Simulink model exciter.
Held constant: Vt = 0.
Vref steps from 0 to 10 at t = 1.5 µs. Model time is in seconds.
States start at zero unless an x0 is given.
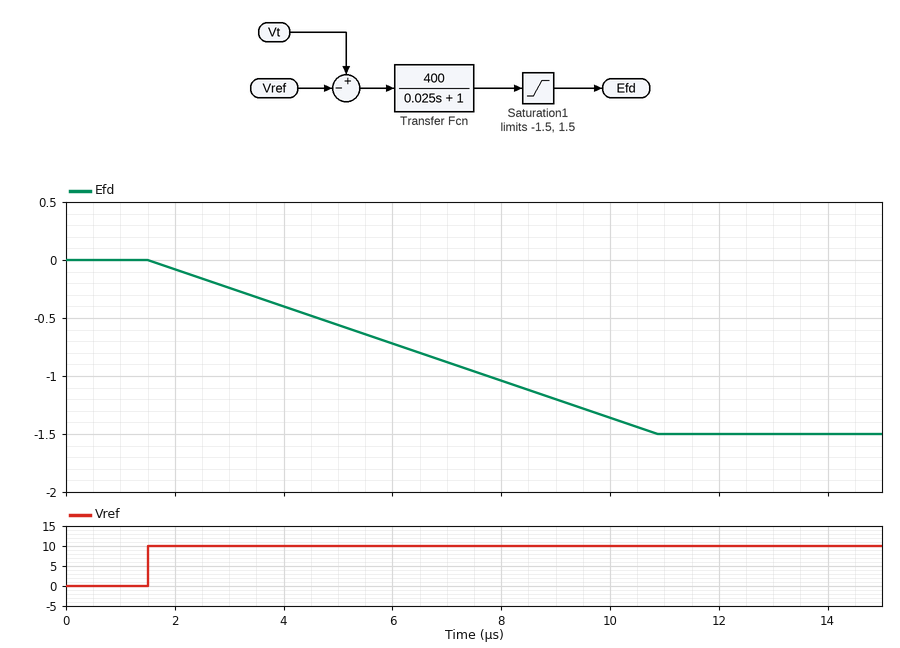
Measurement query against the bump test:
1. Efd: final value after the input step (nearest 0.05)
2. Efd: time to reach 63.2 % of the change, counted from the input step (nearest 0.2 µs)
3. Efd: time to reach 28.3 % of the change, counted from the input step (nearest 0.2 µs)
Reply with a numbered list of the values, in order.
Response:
1. -1.50
2. 6.0 µs
3. 2.6 µs
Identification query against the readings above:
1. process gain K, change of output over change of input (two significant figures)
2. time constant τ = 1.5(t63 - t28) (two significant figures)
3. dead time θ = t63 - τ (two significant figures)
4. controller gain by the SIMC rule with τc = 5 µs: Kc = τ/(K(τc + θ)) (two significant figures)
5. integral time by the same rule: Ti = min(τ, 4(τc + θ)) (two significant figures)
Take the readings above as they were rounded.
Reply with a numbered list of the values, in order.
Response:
1. -0.15
2. 5.1 µs
3. 0.90 µs
4. -5.8
5. 5.1 µs
